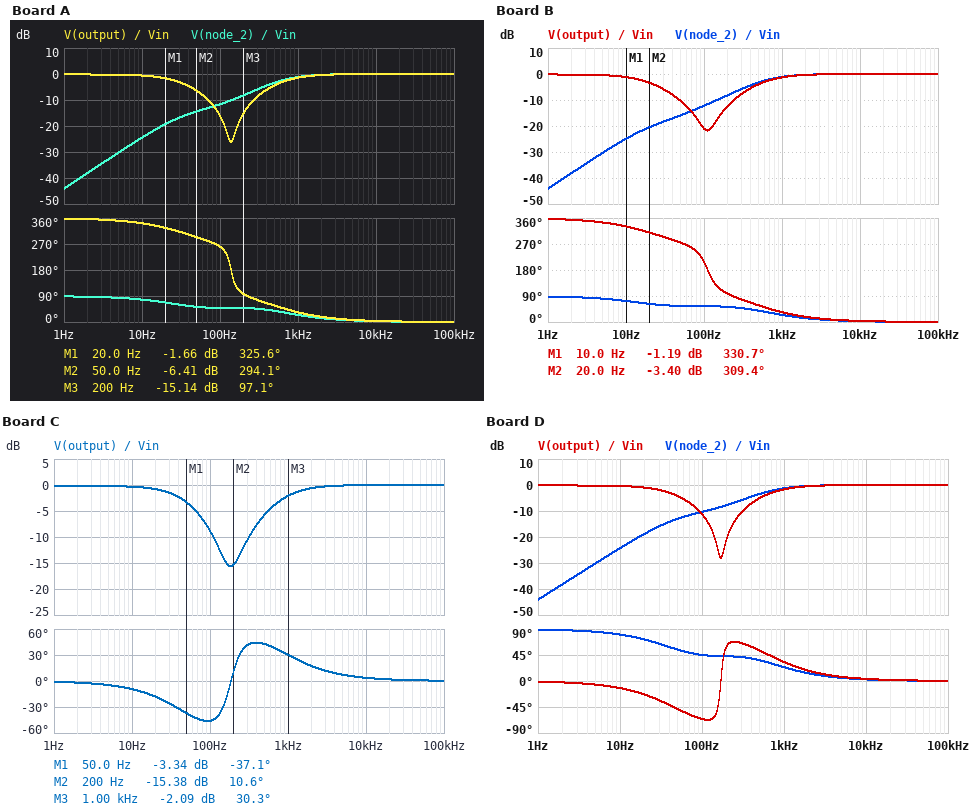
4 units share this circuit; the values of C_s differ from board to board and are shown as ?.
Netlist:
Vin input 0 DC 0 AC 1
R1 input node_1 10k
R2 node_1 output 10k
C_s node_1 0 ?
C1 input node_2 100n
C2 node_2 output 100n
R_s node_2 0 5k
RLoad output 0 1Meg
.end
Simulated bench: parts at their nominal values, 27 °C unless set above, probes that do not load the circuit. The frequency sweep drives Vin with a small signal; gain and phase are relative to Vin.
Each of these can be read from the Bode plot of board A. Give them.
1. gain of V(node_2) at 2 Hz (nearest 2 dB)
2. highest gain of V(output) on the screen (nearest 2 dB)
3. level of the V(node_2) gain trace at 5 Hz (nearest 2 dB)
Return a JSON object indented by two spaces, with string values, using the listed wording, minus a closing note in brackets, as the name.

{
  "gain of V(node_2) at 2 Hz": "-38 dB",
  "highest gain of V(output) on the screen": "0 dB",
  "level of the V(node_2) gain trace at 5 Hz": "-30 dB"
}
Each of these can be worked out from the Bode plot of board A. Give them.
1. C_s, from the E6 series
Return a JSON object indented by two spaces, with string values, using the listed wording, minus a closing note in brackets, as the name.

{
  "C_s, from the E6 series": "330 nF"
}
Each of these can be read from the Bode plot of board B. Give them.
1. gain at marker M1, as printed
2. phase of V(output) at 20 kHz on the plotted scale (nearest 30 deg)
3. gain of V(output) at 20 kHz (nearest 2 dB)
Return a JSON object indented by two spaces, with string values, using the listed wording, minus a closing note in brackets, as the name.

{
  "gain at marker M1, as printed": "-1.19 dB",
  "phase of V(output) at 20 kHz on the plotted scale": "0 deg",
  "gain of V(output) at 20 kHz": "0 dB"
}
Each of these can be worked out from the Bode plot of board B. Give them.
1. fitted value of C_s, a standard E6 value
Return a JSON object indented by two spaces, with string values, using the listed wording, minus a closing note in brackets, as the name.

{
  "fitted value of C_s, a standard E6 value": "680 nF"
}
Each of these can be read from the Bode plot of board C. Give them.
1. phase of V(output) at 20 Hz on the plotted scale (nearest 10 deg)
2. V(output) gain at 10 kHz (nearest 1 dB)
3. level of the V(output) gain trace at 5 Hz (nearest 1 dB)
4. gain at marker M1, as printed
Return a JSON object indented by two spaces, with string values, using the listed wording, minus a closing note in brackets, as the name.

{
  "phase of V(output) at 20 Hz on the plotted scale": "-20 deg",
  "V(output) gain at 10 kHz": "0 dB",
  "level of the V(output) gain trace at 5 Hz": "0 dB",
  "gain at marker M1, as printed": "-3.34 dB"
}
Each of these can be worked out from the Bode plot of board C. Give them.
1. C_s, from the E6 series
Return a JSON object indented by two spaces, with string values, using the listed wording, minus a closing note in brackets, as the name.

{
  "C_s, from the E6 series": "68 nF"
}
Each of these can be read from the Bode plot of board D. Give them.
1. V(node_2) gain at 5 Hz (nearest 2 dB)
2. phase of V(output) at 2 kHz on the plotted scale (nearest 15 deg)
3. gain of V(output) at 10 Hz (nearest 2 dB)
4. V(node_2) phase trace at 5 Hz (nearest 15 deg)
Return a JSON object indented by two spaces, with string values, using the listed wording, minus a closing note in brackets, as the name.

{
  "V(node_2) gain at 5 Hz": "-30 dB",
  "phase of V(output) at 2 kHz on the plotted scale": "15 deg",
  "gain of V(output) at 10 Hz": "0 dB",
  "V(node_2) phase trace at 5 Hz": "90 deg"
}
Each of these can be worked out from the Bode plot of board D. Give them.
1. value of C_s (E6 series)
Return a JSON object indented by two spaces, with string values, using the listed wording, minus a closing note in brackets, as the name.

{
  "value of C_s": "150 nF"
}
